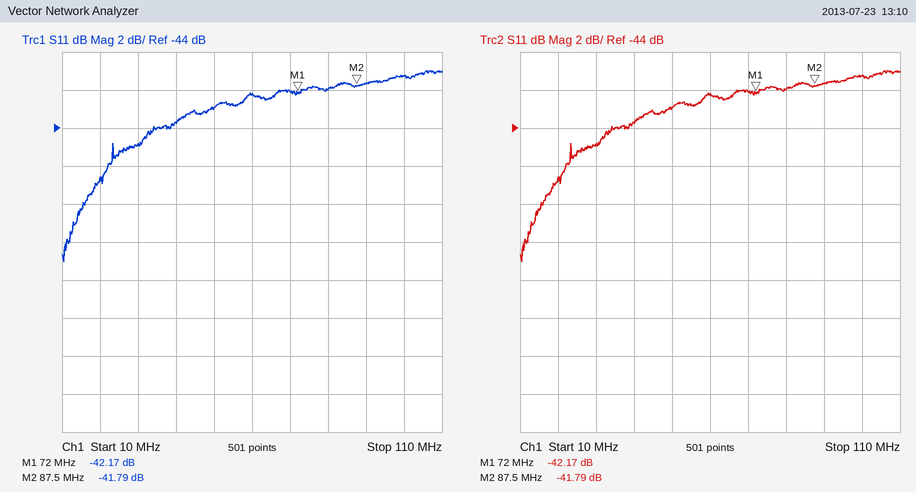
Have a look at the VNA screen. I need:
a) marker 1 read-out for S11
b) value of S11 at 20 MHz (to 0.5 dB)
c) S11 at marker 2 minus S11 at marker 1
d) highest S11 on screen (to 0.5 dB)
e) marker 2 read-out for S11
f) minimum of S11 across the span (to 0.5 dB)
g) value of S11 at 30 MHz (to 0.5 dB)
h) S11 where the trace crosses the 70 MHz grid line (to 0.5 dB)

-42.17 dB
-46.5 dB
0.38 dB
-41.0 dB
-41.79 dB
-51.0 dB
-45.0 dB
-42.0 dB
